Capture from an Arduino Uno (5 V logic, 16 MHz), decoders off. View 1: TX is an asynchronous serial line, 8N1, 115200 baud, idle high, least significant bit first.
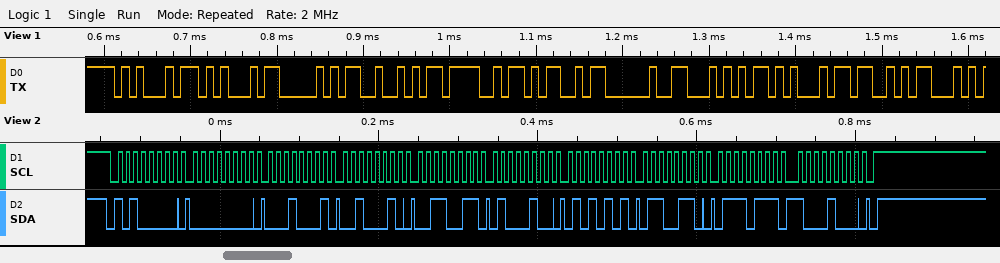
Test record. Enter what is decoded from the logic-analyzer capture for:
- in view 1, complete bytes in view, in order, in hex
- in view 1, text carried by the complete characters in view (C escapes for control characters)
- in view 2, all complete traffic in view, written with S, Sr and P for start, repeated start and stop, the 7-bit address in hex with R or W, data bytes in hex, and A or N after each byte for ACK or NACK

45 45 50 52 4F 4D 20 54 45 53
"EEPROM TES"
S 50W A 00 A 11 A 22 A 33 A 44 A 55 A 66 A 77 A 88 A P
